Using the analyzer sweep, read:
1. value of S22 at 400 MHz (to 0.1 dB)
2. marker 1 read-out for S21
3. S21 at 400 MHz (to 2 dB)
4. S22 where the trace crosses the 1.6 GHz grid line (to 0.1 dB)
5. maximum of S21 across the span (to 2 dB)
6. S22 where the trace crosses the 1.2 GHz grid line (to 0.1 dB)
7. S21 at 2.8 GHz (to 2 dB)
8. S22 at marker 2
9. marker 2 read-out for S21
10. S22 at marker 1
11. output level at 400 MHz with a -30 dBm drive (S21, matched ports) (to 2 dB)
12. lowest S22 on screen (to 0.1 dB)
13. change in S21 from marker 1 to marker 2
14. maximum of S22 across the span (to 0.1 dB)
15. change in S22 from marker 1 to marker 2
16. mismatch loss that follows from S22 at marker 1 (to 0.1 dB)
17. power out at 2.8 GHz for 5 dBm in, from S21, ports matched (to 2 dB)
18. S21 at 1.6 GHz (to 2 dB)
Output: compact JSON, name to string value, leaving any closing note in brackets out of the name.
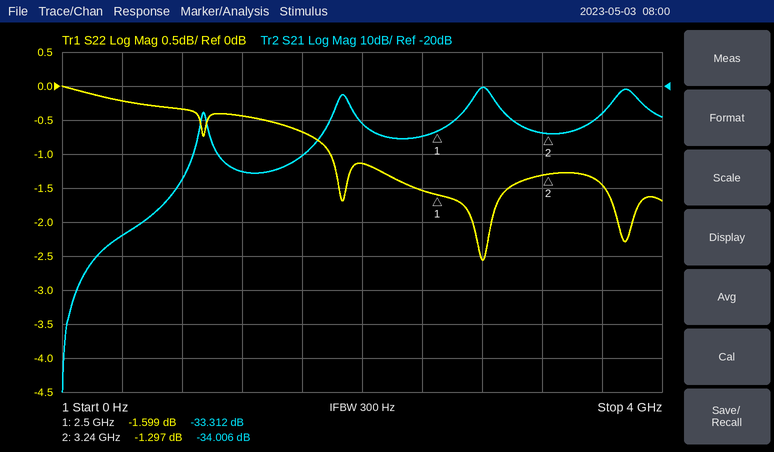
{"value of S22 at 400 MHz": "-0.2 dB", "marker 1 read-out for S21": "-33.312 dB", "S21 at 400 MHz": "-64 dB", "S22 where the trace crosses the 1.6 GHz grid line": "-0.7 dB", "maximum of S21 across the span": "-20 dB", "S22 where the trace crosses the 1.2 GHz grid line": "-0.4 dB", "S21 at 2.8 GHz": "-20 dB", "S22 at marker 2": "-1.297 dB", "marker 2 read-out for S21": "-34.006 dB", "S22 at marker 1": "-1.599 dB", "output level at 400 MHz with a -30 dBm drive (S21, matched ports)": "-94 dBm", "lowest S22 on screen": "-2.6 dB", "change in S21 from marker 1 to marker 2": "-0.694 dB", "maximum of S22 across the span": "0.0 dB", "change in S22 from marker 1 to marker 2": "0.302 dB", "mismatch loss that follows from S22 at marker 1": "5.1 dB", "power out at 2.8 GHz for 5 dBm in, from S21, ports matched": "-16 dBm", "S21 at 1.6 GHz": "-40 dB"}
